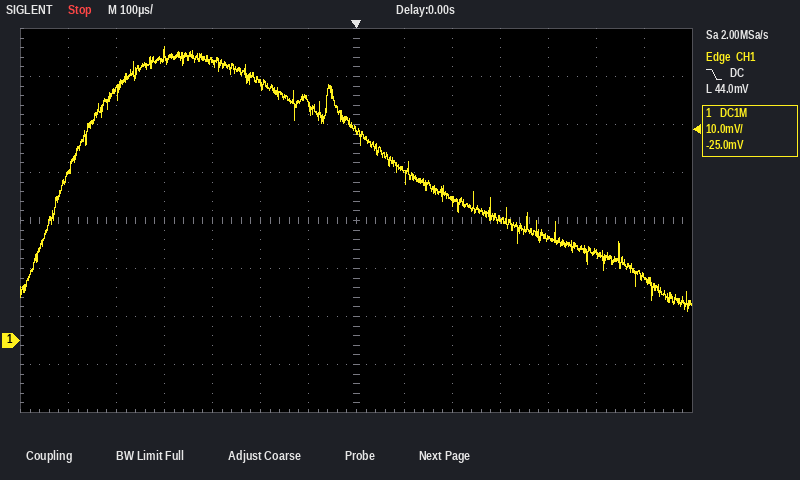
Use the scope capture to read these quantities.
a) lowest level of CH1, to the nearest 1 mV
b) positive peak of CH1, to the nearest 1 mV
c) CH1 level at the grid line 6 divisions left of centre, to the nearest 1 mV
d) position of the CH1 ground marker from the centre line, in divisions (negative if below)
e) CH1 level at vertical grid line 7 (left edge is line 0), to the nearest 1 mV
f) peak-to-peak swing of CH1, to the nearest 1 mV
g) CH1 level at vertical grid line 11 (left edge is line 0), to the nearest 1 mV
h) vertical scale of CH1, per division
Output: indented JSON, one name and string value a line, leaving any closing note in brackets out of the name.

{
  "lowest level of CH1, to the nearest 1 mV": "6 mV",
  "positive peak of CH1, to the nearest 1 mV": "61 mV",
  "CH1 level at the grid line 6 divisions left of centre, to the nearest 1 mV": "35 mV",
  "position of the CH1 ground marker from the centre line, in divisions": "-2.5 div",
  "CH1 level at vertical grid line 7 (left edge is line 0), to the nearest 1 mV": "44 mV",
  "peak-to-peak swing of CH1, to the nearest 1 mV": "55 mV",
  "CH1 level at vertical grid line 11 (left edge is line 0), to the nearest 1 mV": "21 mV",
  "vertical scale of CH1, per division": "10 mV"
}
